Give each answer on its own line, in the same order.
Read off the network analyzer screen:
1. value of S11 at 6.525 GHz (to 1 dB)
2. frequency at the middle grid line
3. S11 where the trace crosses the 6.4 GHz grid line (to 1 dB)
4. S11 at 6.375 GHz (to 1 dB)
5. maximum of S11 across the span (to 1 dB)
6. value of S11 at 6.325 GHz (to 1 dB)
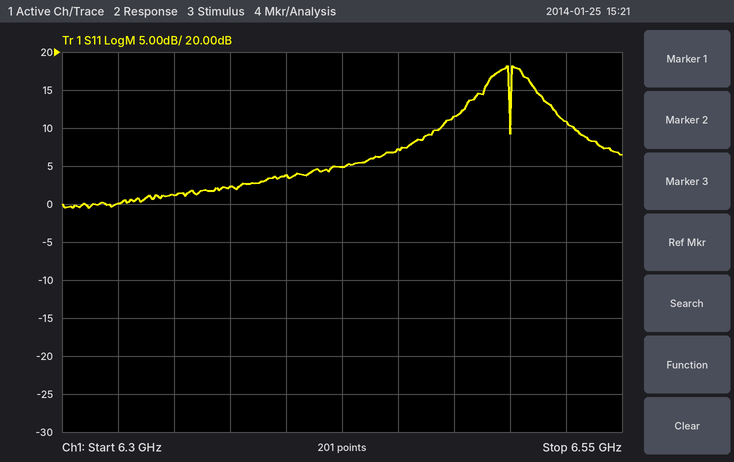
11 dB
6.425 GHz
4 dB
2 dB
18 dB
0 dB
